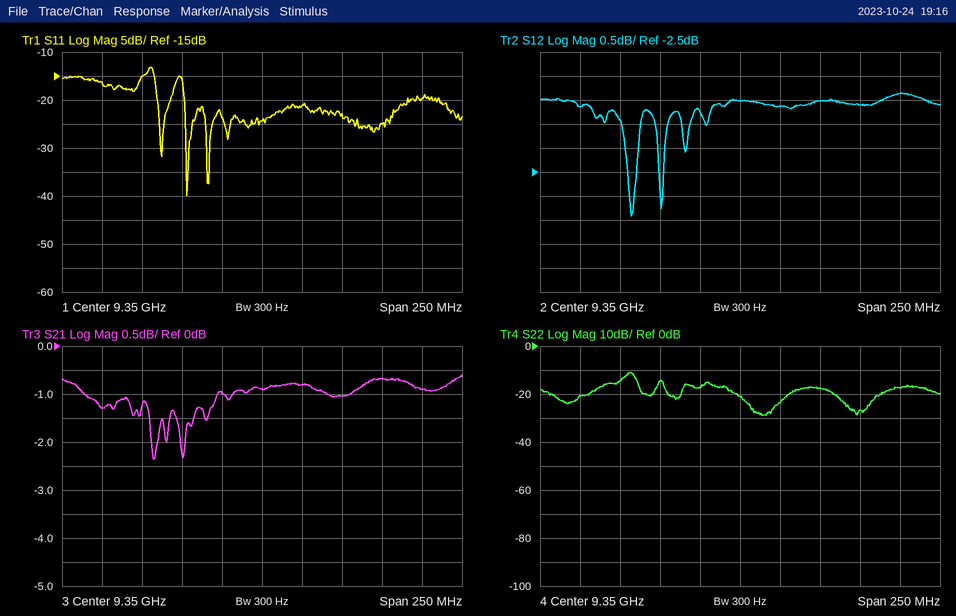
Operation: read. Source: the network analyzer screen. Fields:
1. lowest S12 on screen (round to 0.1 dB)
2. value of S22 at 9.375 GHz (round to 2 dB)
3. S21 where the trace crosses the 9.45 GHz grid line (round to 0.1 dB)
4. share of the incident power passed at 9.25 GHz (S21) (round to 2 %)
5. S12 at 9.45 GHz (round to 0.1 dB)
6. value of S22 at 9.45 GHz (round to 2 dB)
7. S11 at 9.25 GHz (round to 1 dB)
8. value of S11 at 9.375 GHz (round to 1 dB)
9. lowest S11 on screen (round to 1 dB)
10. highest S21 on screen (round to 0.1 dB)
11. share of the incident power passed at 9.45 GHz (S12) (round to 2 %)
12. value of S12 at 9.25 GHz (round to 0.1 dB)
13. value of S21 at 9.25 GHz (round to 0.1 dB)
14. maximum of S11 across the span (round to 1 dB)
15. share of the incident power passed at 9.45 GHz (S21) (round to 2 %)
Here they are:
-3.4 dB
-24 dB
-0.9 dB
74 %
-0.9 dB
-18 dB
-16 dB
-21 dB
-40 dB
-0.6 dB
82 %
-1.1 dB
-1.3 dB
-13 dB
82 %
